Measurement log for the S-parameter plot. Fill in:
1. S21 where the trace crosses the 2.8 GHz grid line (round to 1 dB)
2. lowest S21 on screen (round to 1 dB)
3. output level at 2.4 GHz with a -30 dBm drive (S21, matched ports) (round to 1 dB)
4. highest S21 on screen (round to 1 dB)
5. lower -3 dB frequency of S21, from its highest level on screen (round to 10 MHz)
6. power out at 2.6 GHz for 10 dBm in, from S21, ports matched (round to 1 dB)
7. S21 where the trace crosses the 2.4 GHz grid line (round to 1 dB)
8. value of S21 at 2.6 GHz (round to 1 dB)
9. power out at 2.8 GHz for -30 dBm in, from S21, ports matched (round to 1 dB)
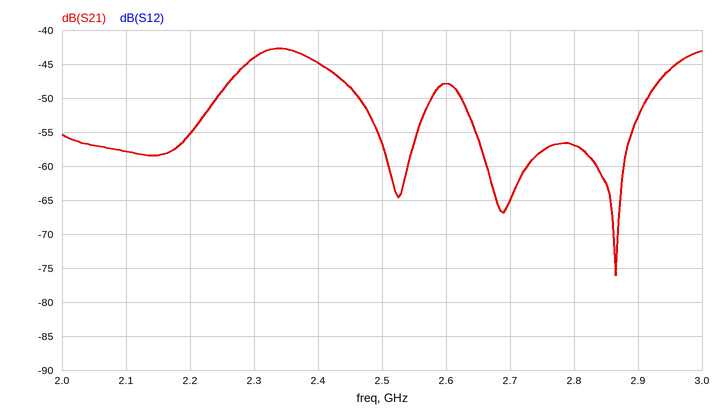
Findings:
-57 dB
-76 dB
-75 dBm
-43 dB
2.28 GHz
-38 dBm
-45 dB
-48 dB
-87 dBm
